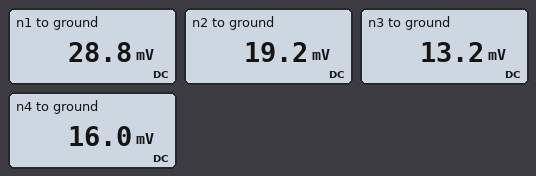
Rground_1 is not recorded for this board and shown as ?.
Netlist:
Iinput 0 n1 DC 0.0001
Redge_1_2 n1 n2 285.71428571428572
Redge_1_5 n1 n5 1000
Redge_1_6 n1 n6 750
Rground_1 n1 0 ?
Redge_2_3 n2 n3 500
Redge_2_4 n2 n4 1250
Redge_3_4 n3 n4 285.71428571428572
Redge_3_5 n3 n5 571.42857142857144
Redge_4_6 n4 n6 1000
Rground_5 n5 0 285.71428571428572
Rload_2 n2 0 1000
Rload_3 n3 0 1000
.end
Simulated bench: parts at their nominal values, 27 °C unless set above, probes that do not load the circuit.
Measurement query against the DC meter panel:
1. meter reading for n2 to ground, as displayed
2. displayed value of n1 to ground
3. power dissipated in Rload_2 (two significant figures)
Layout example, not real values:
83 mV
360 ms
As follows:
19.2 mV
28.8 mV
370 nW
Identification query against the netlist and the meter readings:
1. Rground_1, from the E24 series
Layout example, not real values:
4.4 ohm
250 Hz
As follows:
750 Ω
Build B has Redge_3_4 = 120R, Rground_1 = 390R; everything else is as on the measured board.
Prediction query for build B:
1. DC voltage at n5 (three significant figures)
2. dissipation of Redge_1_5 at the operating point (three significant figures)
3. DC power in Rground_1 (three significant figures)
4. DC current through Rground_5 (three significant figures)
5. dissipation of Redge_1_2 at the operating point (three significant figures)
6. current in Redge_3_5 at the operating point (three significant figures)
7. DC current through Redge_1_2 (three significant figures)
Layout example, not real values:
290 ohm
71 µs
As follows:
6.18 mV
225 nW
1.15 µW
21.6 µA
176 nW
6.62 µA
24.8 µA
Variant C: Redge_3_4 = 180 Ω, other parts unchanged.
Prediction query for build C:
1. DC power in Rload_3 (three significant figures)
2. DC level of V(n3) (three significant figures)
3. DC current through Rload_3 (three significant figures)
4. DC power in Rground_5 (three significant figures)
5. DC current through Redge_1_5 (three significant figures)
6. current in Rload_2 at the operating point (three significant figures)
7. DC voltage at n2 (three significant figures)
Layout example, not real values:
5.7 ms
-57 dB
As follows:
179 nW
13.4 mV
13.4 µA
244 nW
20.4 µA
19.1 µA
19.1 mV
